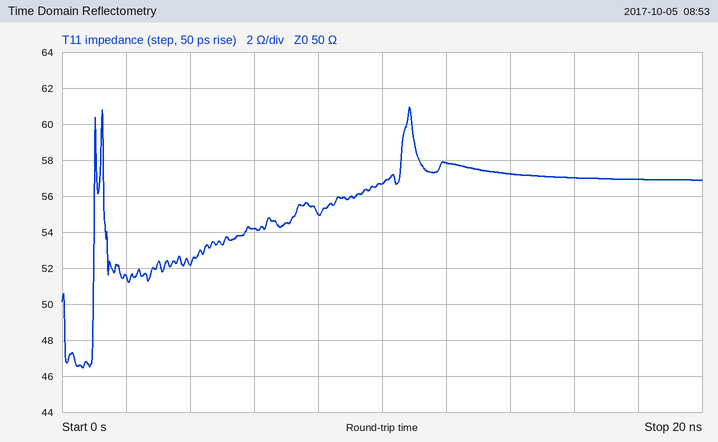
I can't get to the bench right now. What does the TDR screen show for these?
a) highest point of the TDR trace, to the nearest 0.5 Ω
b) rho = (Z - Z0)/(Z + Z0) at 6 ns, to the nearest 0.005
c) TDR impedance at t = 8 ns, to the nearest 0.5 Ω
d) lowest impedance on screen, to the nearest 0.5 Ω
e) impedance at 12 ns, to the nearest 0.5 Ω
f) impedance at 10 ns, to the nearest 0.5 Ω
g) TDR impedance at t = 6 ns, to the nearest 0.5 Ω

61.0 Ω
+0.040
55.0 Ω
46.5 Ω
58.0 Ω
56.5 Ω
54.0 Ω
